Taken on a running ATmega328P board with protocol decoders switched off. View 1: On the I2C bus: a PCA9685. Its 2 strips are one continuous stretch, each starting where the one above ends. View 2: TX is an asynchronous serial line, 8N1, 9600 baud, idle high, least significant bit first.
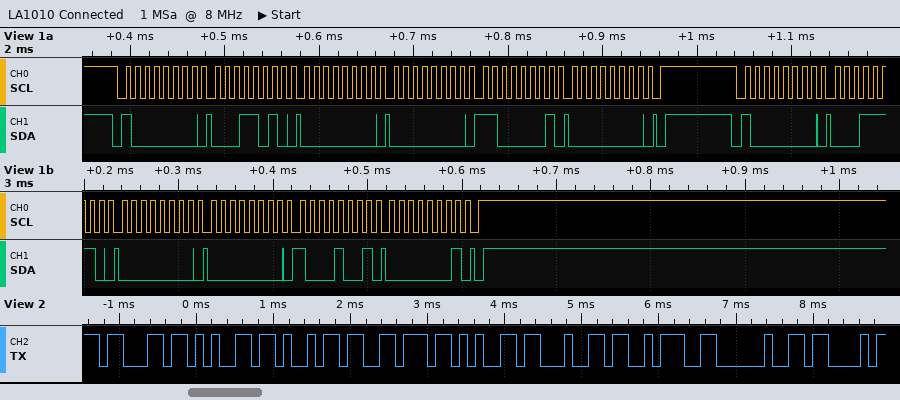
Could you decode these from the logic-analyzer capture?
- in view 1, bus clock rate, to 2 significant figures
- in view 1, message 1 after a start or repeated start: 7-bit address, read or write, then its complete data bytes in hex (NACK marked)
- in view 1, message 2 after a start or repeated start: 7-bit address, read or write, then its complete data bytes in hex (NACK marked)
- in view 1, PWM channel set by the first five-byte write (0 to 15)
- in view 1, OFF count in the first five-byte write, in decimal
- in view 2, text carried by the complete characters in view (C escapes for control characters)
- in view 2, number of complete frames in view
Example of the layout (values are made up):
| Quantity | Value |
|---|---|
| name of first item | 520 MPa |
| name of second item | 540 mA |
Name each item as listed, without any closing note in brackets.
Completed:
| Quantity | Value |
|---|---|
| in view 1, bus clock rate, to 2 significant figures | 100 kHz |
| in view 1, message 1 after a start or repeated start: 7-bit address, read or write, then its complete data bytes in hex | 0x40 write: 1A 00 00 C1 00 |
| in view 1, message 2 after a start or repeated start: 7-bit address, read or write, then its complete data bytes in hex | 0x40 write: 1E 00 00 89 01 |
| in view 1, PWM channel set by the first five-byte write | 5 |
| in view 1, OFF count in the first five-byte write, in decimal | 193 |
| in view 2, text carried by the complete characters in view | "ceived: C" |
| in view 2, number of complete frames in view | 9 |
